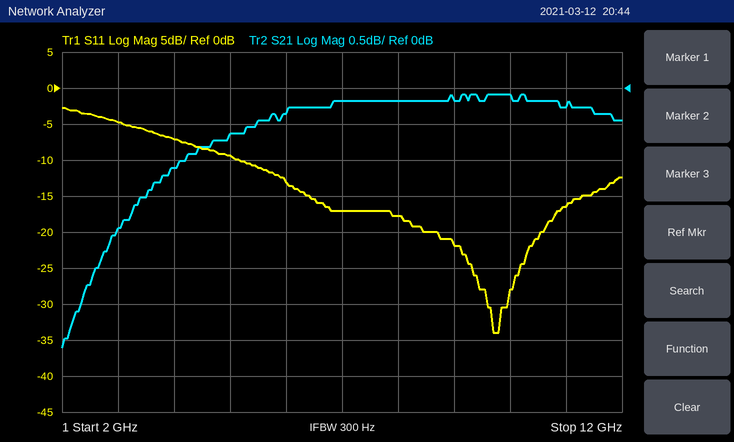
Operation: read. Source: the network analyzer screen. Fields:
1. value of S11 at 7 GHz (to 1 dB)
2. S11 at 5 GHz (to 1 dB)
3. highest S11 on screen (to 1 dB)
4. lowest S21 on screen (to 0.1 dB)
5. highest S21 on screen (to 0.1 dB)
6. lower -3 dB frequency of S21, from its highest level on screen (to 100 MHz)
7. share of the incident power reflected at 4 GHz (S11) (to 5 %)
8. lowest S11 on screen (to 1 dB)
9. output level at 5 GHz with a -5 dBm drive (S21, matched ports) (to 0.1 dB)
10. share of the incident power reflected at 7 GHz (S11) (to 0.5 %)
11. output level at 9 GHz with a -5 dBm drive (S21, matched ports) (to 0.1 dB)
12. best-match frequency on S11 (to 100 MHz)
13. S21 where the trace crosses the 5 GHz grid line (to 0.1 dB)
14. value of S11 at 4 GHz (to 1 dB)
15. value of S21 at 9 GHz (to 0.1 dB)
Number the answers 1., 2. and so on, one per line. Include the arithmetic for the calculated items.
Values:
1. -17 dB
2. -9 dB
3. -3 dB
4. -3.6 dB
5. -0.1 dB
6. 2.3 GHz
7. 10^(-7/10) ≈ 20 %
8. -34 dB
9. -5 dBm + (-0.6 dB) = -5.6 dBm
10. 10^(-17/10) ≈ 2.0 %
11. -5 dBm + (-0.2 dB) = -5.2 dBm
12. 9.7 GHz
13. -0.6 dB
14. -7 dB
15. -0.2 dB
